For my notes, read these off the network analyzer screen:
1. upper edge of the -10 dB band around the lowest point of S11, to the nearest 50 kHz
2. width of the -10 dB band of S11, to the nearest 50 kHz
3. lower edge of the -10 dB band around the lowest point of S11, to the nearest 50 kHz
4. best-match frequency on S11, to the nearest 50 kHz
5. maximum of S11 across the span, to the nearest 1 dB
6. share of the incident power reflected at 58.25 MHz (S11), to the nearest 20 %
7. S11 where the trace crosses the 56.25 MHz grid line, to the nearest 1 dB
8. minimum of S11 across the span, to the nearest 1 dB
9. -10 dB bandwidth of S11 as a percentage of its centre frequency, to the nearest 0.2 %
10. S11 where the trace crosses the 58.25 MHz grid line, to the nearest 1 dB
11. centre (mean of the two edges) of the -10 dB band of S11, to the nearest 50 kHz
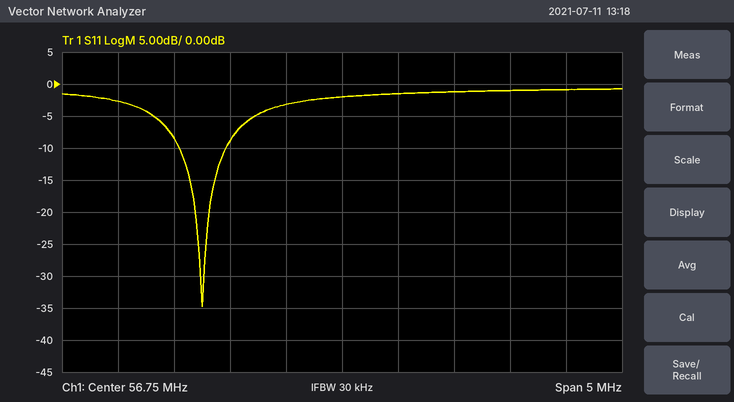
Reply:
55.70 MHz
400 kHz
55.30 MHz
55.50 MHz
-1 dB
80 %
-3 dB
-35 dB
0.8 %
-1 dB
55.50 MHz
